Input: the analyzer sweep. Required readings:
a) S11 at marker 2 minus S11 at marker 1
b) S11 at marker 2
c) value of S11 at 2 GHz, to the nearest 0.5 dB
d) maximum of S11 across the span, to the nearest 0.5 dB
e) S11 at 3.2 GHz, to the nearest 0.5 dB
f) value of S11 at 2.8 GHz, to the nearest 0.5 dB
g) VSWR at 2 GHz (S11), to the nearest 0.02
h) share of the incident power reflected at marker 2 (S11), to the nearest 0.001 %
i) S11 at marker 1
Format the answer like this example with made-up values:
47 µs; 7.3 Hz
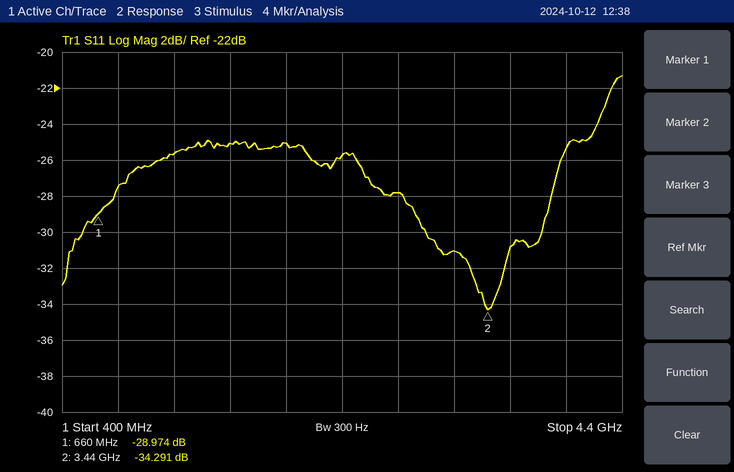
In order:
-5.317 dB; -34.291 dB; -25.0 dB; -21.5 dB; -31.0 dB; -28.0 dB; 1.12; 0.037 %; -28.974 dB
